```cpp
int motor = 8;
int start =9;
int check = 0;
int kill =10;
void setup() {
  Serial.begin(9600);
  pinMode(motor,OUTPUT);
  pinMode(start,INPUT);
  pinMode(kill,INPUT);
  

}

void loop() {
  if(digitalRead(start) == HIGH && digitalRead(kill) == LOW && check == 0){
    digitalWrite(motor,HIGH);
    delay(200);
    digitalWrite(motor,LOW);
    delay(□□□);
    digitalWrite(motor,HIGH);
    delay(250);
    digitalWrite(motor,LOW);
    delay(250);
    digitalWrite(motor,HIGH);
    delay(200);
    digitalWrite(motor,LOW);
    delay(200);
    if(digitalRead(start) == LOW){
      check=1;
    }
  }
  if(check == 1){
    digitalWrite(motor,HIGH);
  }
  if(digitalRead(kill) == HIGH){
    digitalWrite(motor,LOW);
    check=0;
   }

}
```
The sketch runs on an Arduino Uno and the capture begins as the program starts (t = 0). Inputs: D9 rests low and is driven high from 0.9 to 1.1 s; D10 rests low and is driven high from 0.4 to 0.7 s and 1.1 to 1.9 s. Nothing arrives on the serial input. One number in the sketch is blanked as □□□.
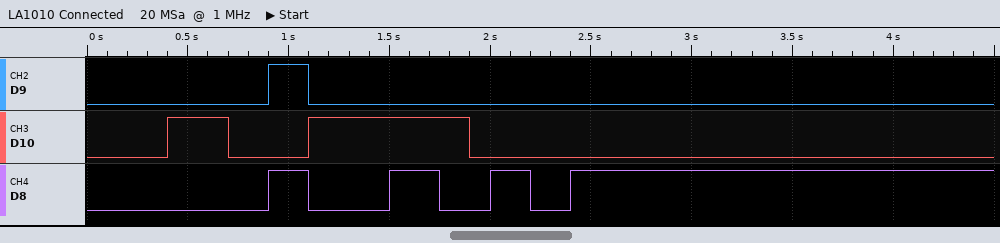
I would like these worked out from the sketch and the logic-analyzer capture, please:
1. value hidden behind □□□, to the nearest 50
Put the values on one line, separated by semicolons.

400
